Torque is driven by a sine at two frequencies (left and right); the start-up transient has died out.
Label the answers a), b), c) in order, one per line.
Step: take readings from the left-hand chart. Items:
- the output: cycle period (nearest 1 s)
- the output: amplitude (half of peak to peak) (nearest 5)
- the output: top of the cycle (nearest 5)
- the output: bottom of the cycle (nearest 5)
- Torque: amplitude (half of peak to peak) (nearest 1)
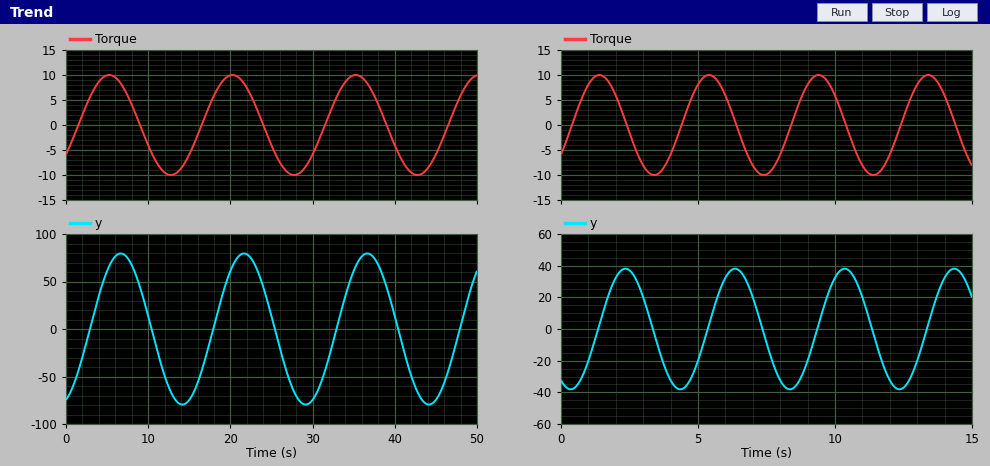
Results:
a) 15 s
b) 80
c) 80
d) -80
e) 10
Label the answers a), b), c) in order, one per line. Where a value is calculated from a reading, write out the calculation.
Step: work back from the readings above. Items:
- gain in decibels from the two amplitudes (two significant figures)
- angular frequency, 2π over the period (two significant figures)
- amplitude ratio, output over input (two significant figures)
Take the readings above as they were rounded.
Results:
a) 20 log10(80 / 10) = 18 dB
b) 2π / 15 = 0.42 rad/s
c) 80 / 10 = 8.0
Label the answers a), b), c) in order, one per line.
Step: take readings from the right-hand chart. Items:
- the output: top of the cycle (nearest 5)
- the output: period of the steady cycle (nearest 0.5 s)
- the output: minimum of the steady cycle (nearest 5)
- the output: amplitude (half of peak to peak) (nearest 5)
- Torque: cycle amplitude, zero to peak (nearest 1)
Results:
a) 40
b) 4.0 s
c) -40
d) 40
e) 10
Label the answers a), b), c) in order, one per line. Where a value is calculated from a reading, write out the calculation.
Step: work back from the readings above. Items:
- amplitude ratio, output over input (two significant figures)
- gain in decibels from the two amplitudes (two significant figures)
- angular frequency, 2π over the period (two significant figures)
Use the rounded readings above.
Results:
a) 40 / 10 = 4.0
b) 20 log10(40 / 10) = 12 dB
c) 2π / 4 = 1.6 rad/s
